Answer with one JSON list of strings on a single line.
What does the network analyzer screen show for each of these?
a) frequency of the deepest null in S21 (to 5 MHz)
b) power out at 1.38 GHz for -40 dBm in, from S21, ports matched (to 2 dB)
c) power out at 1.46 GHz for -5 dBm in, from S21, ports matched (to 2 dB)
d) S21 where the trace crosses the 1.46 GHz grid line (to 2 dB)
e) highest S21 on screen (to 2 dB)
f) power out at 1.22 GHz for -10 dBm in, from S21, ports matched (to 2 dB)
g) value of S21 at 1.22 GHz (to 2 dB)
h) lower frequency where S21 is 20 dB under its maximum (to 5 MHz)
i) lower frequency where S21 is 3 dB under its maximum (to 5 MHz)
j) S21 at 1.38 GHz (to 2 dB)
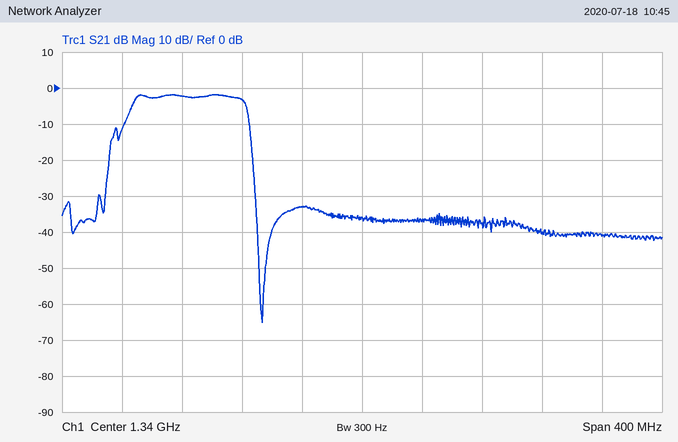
["1.275 GHz", "-76 dBm", "-46 dBm", "-40 dB", "-2 dB", "-12 dBm", "-2 dB", "1.170 GHz", "1.185 GHz", "-36 dB"]
